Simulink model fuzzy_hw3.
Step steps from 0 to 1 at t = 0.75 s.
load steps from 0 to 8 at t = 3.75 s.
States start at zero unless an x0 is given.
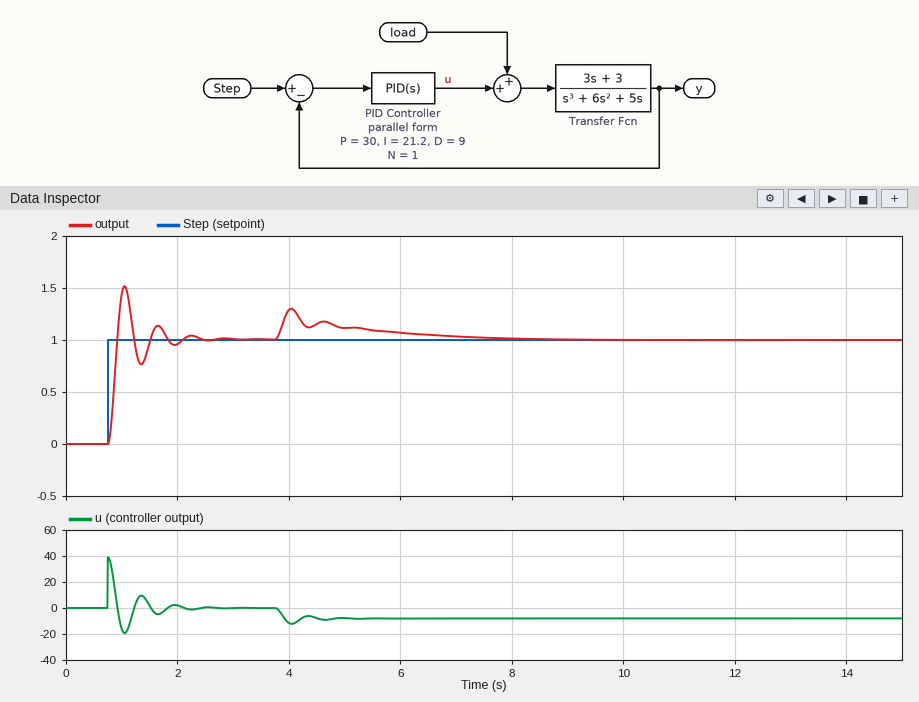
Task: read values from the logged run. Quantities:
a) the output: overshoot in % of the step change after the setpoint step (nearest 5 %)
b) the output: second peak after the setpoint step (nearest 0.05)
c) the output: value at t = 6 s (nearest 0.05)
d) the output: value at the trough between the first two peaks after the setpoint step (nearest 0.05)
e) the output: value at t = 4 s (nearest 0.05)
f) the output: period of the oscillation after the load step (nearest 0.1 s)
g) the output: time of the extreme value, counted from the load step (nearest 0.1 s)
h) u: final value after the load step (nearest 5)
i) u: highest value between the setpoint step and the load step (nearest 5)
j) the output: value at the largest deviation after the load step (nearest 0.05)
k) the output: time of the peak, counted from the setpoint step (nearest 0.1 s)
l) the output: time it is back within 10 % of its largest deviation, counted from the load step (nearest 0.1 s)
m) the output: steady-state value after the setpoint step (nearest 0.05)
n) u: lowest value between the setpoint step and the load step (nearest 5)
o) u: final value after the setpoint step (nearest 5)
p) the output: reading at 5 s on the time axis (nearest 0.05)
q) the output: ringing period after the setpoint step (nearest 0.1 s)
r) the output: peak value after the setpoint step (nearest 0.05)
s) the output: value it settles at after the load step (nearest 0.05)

50 %
1.15
1.05
0.75
1.30
0.6 s
0.3 s
-10
40
1.30
0.3 s
3.4 s
1.00
-20
0
1.10
0.6 s
1.50
1.00
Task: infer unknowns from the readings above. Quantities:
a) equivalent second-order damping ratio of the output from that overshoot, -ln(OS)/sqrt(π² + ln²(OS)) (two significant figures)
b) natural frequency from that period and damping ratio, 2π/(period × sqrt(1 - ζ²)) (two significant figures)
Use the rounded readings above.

0.22
11 rad/s
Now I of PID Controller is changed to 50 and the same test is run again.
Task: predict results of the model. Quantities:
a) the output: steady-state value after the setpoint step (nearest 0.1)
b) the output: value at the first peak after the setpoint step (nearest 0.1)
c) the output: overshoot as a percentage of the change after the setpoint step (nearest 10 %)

1.0
1.6
60 %
